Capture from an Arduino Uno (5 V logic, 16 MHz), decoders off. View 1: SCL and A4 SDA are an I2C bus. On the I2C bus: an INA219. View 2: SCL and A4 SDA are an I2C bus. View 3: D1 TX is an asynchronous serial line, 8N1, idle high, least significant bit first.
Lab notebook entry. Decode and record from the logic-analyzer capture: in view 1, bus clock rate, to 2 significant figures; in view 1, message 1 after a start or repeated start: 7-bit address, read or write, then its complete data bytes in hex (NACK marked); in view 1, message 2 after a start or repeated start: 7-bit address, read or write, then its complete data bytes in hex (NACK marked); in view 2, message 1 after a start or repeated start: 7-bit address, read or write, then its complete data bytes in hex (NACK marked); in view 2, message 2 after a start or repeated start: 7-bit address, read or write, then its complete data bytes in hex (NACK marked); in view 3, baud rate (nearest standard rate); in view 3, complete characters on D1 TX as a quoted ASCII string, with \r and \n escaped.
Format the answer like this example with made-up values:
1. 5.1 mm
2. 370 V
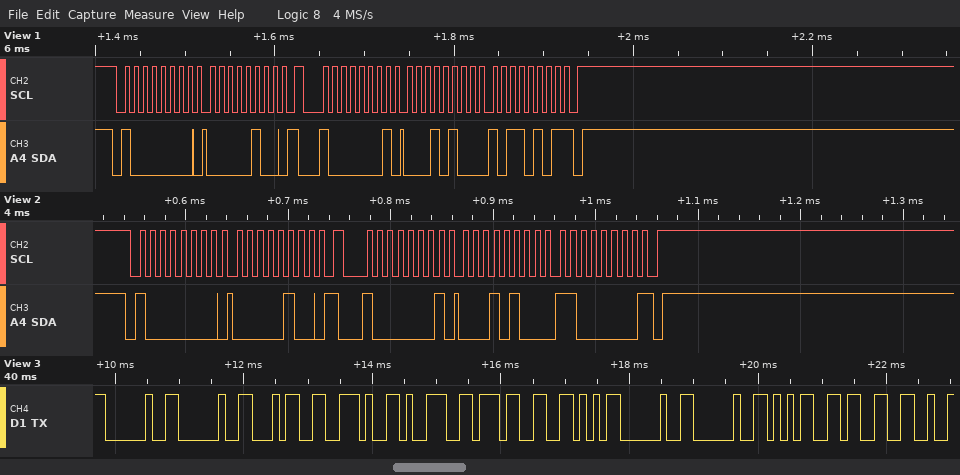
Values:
1. 100 kHz
2. 0x40 write: 04
3. 0x40 read: 14 B5 NACK
4. 0x40 write: 04
5. 0x40 read: 14 C0 NACK
6. 9600 baud
7. "  4.97V  53"
